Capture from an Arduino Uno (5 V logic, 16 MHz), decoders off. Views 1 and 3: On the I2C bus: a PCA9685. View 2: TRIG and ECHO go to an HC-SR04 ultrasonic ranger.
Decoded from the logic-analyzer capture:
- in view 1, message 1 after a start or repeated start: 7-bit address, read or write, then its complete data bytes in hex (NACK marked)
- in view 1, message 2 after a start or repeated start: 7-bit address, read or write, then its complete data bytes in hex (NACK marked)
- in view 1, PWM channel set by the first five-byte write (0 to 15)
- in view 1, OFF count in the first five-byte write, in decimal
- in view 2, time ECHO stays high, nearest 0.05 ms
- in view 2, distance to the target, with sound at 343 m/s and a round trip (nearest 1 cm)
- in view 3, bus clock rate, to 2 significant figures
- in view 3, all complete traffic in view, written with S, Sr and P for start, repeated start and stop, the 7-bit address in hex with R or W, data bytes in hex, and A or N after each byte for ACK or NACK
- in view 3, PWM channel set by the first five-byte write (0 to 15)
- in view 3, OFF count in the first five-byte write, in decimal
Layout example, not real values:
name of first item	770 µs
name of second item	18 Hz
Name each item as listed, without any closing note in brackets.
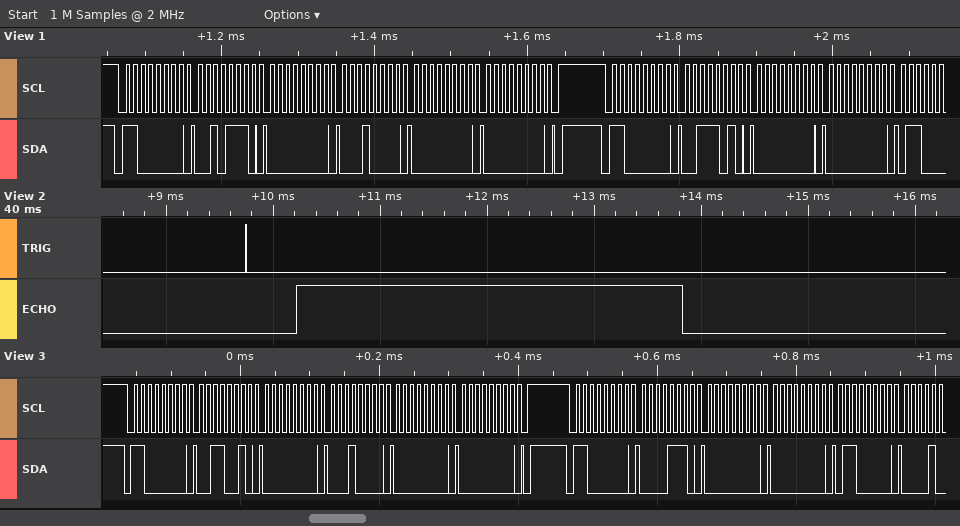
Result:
in view 1, message 1 after a start or repeated start: 7-bit address, read or write, then its complete data bytes in hex	0x60 write: 2E 00 10 00 00
in view 1, message 2 after a start or repeated start: 7-bit address, read or write, then its complete data bytes in hex	0x60 write: 3A 00 00
in view 1, PWM channel set by the first five-byte write	10
in view 1, OFF count in the first five-byte write, in decimal	0
in view 2, time ECHO stays high, nearest 0.05 ms	3.60 ms
in view 2, distance to the target, with sound at 343 m/s and a round trip	62 cm
in view 3, bus clock rate, to 2 significant figures	100 kHz
in view 3, all complete traffic in view, written with S, Sr and P for start, repeated start and stop, the 7-bit address in hex with R or W, data bytes in hex, and A or N after each byte for ACK or NACK	S 60W A 32 A 00 A 10 A 00 A 00 A P S 60W A 0E A 00 A 00 A 60 A
in view 3, PWM channel set by the first five-byte write	11
in view 3, OFF count in the first five-byte write, in decimal	0
